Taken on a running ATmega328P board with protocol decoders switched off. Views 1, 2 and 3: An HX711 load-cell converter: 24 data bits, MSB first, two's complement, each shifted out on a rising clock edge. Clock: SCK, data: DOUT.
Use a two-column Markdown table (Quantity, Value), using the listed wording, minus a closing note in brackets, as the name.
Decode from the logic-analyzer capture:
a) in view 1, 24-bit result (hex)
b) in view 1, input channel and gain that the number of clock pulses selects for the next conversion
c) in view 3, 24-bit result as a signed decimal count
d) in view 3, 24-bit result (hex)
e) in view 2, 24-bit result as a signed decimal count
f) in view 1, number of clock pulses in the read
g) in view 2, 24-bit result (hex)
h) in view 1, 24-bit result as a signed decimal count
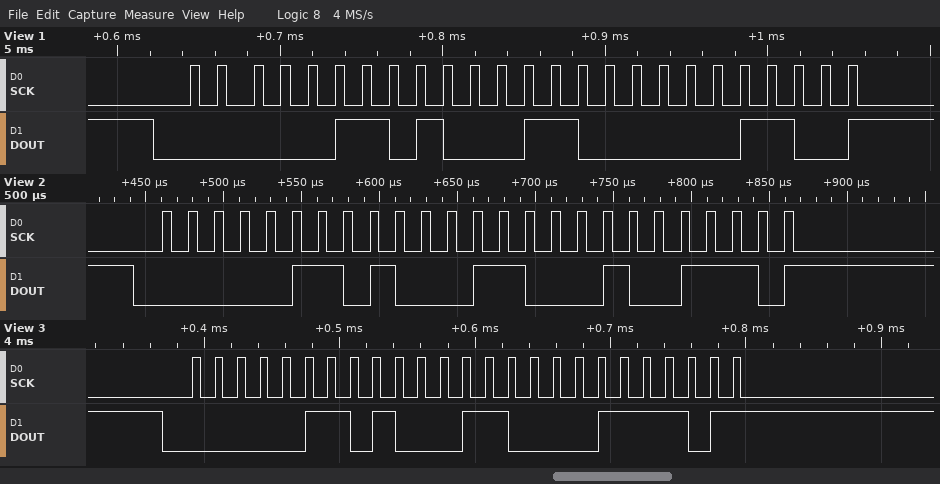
| Quantity | Value |
|---|---|
| in view 1, 24-bit result | 0x068C0C |
| in view 1, input channel and gain that the number of clock pulses selects for the next conversion | channel A, gain 128 |
| in view 3, 24-bit result as a signed decimal count | 429117 |
| in view 3, 24-bit result | 0x068C3D |
| in view 2, 24-bit result as a signed decimal count | 429134 |
| in view 1, number of clock pulses in the read | 25 |
| in view 2, 24-bit result | 0x068C4E |
| in view 1, 24-bit result as a signed decimal count | 429068 |
